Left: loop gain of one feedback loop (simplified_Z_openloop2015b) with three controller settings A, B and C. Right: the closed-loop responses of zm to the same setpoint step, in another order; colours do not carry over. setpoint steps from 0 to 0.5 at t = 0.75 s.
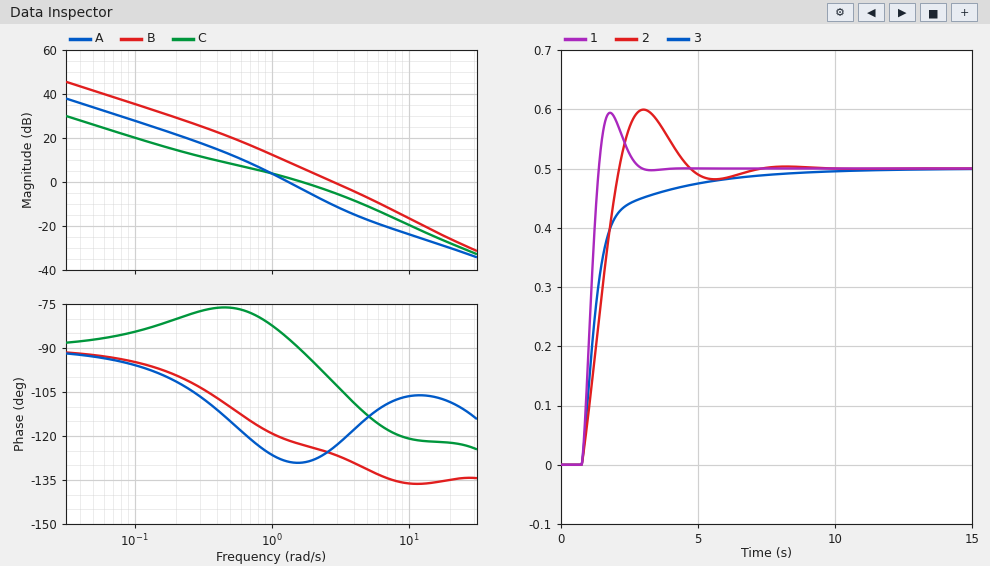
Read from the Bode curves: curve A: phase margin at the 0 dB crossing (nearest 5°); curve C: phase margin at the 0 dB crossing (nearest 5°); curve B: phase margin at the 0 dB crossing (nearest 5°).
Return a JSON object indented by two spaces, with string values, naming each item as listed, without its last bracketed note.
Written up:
{
  "curve A: phase margin at the 0 dB crossing": "50°",
  "curve C: phase margin at the 0 dB crossing": "90°",
  "curve B: phase margin at the 0 dB crossing": "55°"
}
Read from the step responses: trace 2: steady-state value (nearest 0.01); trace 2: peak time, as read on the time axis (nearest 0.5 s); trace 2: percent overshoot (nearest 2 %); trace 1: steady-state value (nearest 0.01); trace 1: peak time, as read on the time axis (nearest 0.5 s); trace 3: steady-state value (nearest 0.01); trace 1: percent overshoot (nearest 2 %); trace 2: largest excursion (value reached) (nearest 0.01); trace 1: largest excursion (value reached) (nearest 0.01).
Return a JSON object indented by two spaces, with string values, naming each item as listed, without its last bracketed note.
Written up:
{
  "trace 2: steady-state value": "0.50",
  "trace 2: peak time, as read on the time axis": "3.0 s",
  "trace 2: percent overshoot": "20 %",
  "trace 1: steady-state value": "0.50",
  "trace 1: peak time, as read on the time axis": "2.0 s",
  "trace 3: steady-state value": "0.50",
  "trace 1: percent overshoot": "18 %",
  "trace 2: largest excursion (value reached)": "0.60",
  "trace 1: largest excursion (value reached)": "0.59"
}
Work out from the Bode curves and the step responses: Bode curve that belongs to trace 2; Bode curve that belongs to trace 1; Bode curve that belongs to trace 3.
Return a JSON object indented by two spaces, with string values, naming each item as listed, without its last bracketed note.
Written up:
{
  "Bode curve that belongs to trace 2": "A",
  "Bode curve that belongs to trace 1": "B",
  "Bode curve that belongs to trace 3": "C"
}
